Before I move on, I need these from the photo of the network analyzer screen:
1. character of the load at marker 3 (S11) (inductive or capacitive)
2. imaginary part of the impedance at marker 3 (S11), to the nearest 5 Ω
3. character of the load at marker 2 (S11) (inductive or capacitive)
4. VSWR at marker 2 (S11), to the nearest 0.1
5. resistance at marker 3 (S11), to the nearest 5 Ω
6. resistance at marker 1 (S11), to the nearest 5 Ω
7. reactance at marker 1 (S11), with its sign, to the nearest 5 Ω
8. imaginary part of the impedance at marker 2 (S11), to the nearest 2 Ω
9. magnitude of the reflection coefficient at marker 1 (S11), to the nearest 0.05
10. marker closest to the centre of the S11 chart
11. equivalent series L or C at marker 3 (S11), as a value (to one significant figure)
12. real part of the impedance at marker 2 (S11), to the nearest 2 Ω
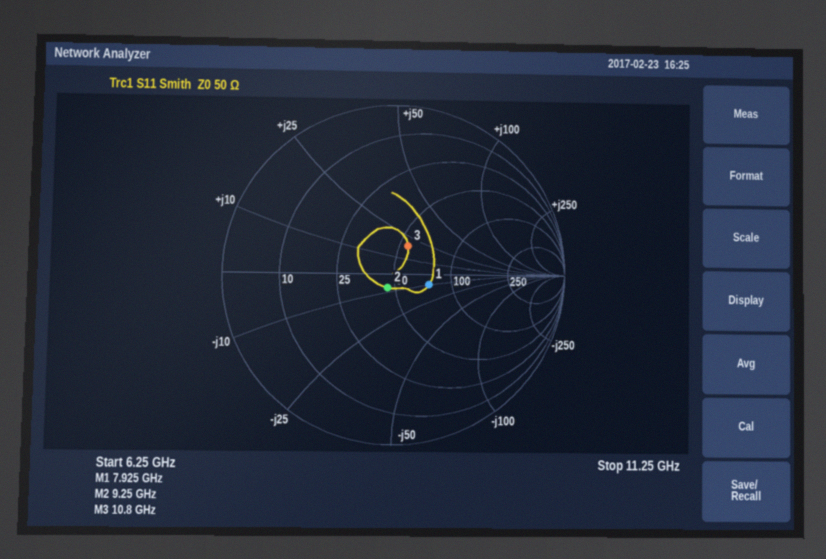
inductive
+20 Ω
capacitive
1.2
55 Ω
75 Ω
-10 Ω
-8 Ω
0.20
marker 2
300 pH
46 Ω
